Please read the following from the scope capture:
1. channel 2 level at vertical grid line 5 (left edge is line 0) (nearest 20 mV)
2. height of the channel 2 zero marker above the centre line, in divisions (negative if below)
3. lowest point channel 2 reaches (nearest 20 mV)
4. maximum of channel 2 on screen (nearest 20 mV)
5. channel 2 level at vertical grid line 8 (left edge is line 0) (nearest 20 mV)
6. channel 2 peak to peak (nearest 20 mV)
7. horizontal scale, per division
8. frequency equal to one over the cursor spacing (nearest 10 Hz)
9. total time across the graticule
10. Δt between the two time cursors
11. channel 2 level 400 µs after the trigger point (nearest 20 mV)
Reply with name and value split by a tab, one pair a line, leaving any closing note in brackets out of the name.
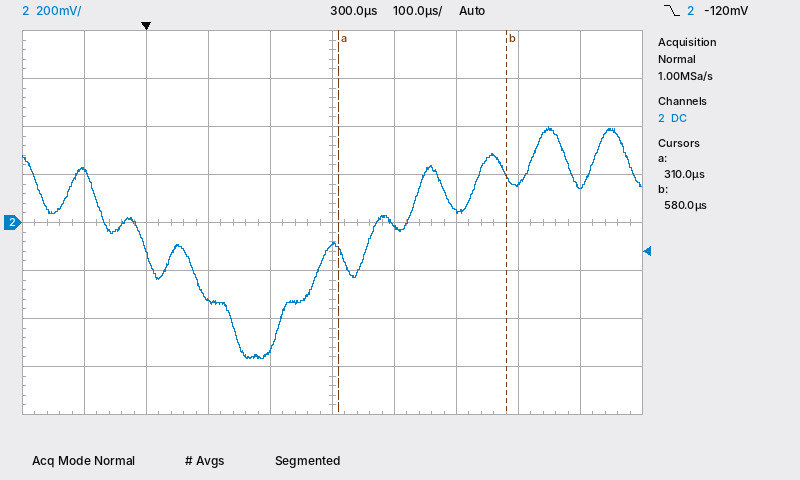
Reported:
channel 2 level at vertical grid line 5 (left edge is line 0)	-100 mV
height of the channel 2 zero marker above the centre line, in divisions	0.0 div
lowest point channel 2 reaches	-560 mV
maximum of channel 2 on screen	400 mV
channel 2 level at vertical grid line 8 (left edge is line 0)	160 mV
channel 2 peak to peak	960 mV
horizontal scale, per division	100 µs
frequency equal to one over the cursor spacing	3.70 kHz
total time across the graticule	1 ms
Δt between the two time cursors	270 µs
channel 2 level 400 µs after the trigger point	-20 mV
